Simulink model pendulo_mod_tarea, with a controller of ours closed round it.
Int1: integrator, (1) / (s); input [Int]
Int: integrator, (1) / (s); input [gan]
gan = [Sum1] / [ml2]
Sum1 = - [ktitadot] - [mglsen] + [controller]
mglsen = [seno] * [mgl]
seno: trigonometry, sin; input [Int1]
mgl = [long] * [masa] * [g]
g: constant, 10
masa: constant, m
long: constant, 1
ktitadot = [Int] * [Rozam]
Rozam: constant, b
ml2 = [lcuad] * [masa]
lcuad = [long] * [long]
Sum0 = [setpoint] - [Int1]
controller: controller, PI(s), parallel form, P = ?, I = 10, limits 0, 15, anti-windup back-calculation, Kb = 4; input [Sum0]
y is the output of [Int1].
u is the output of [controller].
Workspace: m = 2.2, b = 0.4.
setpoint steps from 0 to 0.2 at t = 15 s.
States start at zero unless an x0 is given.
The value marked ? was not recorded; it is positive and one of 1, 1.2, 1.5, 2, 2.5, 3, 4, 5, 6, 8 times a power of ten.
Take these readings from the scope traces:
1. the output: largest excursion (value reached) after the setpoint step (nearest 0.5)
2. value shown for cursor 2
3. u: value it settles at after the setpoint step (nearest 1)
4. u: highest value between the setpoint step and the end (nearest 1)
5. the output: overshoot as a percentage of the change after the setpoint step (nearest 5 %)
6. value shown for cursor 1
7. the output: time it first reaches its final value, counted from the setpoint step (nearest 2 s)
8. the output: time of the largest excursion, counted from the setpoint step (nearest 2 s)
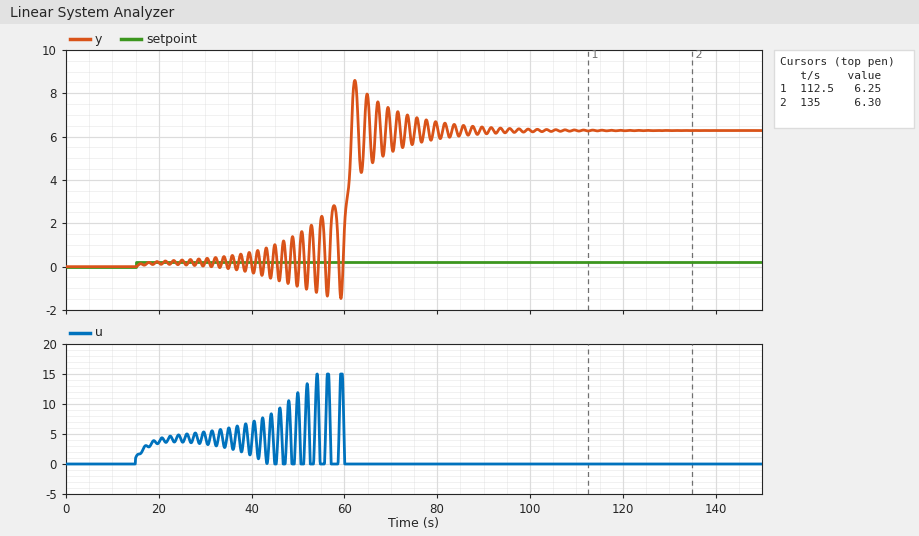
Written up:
8.5
6.30
0
15
35 %
6.25
46 s
48 s
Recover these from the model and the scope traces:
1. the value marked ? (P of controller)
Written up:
5
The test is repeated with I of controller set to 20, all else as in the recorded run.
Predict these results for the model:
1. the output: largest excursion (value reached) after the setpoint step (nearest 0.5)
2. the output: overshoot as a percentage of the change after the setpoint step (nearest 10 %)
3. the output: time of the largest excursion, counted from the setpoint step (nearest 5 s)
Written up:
9.0
40 %
20 s
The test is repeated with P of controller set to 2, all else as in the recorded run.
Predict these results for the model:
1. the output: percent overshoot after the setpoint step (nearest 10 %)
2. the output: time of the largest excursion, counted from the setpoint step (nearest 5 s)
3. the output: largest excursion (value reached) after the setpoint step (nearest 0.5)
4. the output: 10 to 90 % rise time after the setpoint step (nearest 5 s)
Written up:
40 %
35 s
9.0
15 s
